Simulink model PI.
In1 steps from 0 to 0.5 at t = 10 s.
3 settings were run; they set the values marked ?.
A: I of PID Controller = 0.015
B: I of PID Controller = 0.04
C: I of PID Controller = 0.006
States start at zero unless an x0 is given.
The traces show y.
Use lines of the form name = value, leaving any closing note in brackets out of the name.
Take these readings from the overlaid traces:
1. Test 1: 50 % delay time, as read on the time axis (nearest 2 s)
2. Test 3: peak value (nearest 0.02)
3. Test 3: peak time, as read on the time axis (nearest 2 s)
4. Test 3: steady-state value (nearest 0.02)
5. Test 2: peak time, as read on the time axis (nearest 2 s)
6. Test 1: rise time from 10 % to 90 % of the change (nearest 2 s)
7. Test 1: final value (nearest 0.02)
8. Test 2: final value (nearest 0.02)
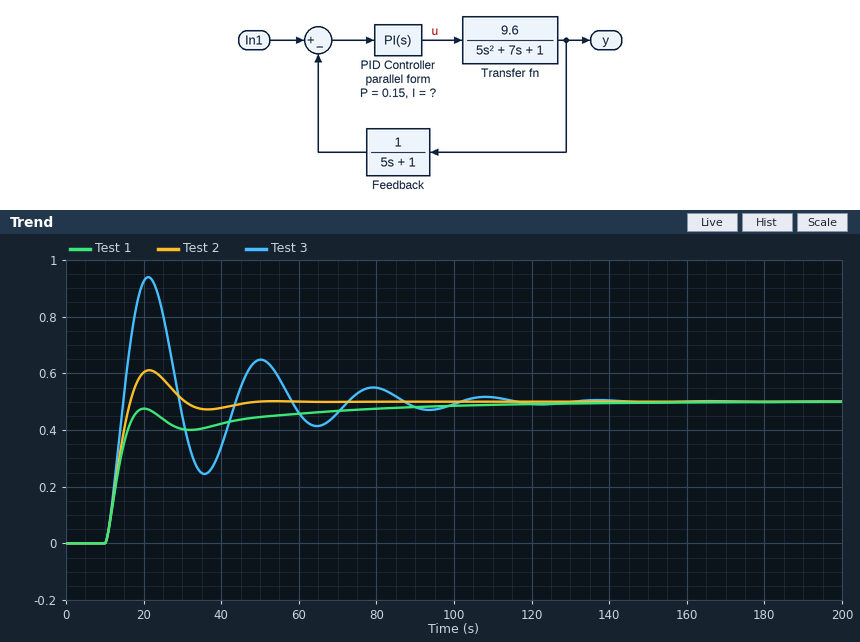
Test 1: 50 % delay time, as read on the time axis = 14 s
Test 3: peak value = 0.94
Test 3: peak time, as read on the time axis = 22 s
Test 3: steady-state value = 0.50
Test 2: peak time, as read on the time axis = 22 s
Test 1: rise time from 10 % to 90 % of the change = 6 s
Test 1: final value = 0.50
Test 2: final value = 0.50
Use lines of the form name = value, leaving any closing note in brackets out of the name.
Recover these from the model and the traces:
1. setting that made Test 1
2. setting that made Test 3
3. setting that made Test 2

setting that made Test 1 = C
setting that made Test 3 = B
setting that made Test 2 = A
